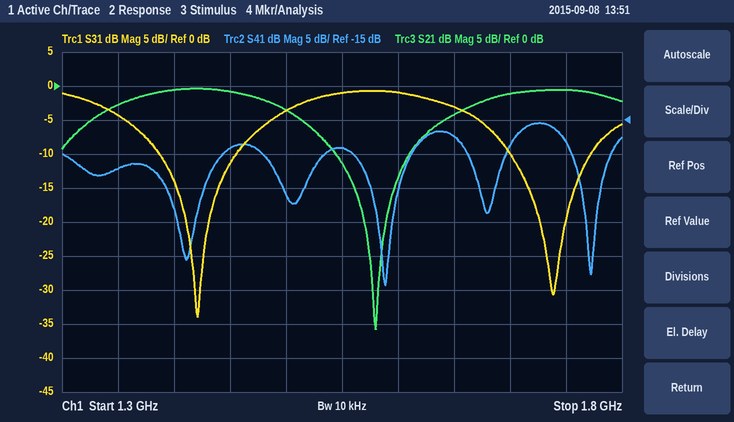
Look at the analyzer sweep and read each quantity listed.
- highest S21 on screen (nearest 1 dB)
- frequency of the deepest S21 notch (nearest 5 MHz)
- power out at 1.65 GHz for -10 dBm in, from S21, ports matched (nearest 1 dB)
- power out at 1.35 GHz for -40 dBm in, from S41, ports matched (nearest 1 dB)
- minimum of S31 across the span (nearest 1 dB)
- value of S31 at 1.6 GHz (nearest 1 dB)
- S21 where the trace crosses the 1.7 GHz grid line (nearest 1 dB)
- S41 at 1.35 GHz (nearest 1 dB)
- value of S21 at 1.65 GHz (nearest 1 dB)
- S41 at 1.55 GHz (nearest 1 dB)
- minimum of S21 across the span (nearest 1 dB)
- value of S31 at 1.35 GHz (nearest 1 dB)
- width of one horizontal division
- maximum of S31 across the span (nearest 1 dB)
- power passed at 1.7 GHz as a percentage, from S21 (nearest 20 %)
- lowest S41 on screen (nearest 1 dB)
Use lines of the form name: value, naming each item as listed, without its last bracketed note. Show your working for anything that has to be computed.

highest S21 on screen: 0 dB
frequency of the deepest S21 notch: 1.580 GHz
power out at 1.65 GHz for -10 dBm in, from S21, ports matched: -10 dBm + (-4 dB) = -14 dBm
power out at 1.35 GHz for -40 dBm in, from S41, ports matched: -40 dBm + (-22 dB) = -62 dBm
minimum of S31 across the span: -34 dB
value of S31 at 1.6 GHz: -1 dB
S21 where the trace crosses the 1.7 GHz grid line: -1 dB
S41 at 1.35 GHz: -22 dB
value of S21 at 1.65 GHz: -4 dB
S41 at 1.55 GHz: -19 dB
minimum of S21 across the span: -36 dB
value of S31 at 1.35 GHz: -4 dB
width of one horizontal division: 50 MHz
maximum of S31 across the span: -1 dB
power passed at 1.7 GHz as a percentage, from S21: 10^(-1/10) ≈ 79.4 %, so 80 % to the nearest 20 %
lowest S41 on screen: -39 dB
